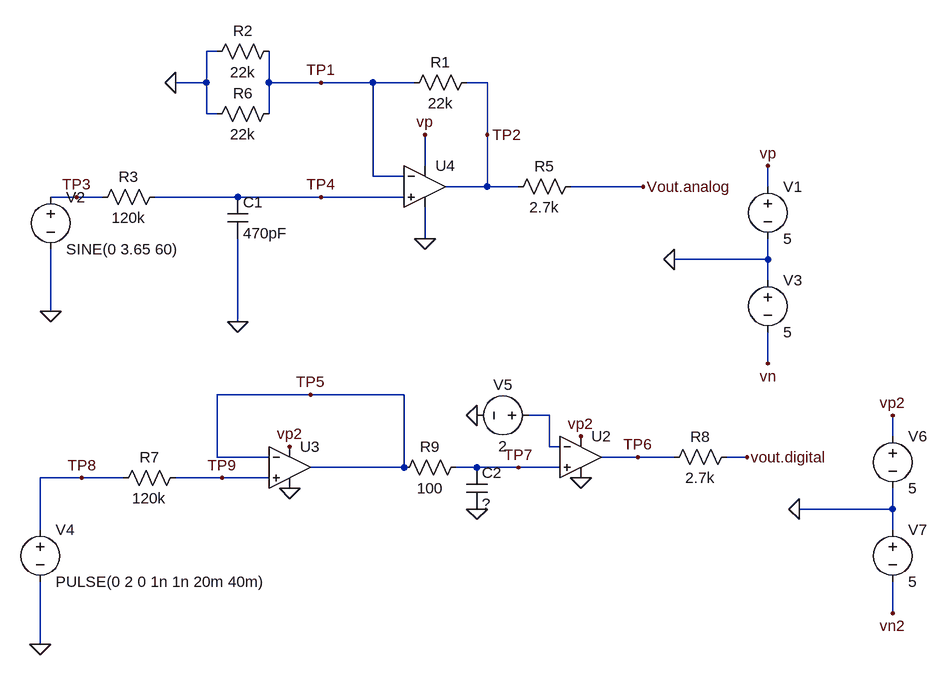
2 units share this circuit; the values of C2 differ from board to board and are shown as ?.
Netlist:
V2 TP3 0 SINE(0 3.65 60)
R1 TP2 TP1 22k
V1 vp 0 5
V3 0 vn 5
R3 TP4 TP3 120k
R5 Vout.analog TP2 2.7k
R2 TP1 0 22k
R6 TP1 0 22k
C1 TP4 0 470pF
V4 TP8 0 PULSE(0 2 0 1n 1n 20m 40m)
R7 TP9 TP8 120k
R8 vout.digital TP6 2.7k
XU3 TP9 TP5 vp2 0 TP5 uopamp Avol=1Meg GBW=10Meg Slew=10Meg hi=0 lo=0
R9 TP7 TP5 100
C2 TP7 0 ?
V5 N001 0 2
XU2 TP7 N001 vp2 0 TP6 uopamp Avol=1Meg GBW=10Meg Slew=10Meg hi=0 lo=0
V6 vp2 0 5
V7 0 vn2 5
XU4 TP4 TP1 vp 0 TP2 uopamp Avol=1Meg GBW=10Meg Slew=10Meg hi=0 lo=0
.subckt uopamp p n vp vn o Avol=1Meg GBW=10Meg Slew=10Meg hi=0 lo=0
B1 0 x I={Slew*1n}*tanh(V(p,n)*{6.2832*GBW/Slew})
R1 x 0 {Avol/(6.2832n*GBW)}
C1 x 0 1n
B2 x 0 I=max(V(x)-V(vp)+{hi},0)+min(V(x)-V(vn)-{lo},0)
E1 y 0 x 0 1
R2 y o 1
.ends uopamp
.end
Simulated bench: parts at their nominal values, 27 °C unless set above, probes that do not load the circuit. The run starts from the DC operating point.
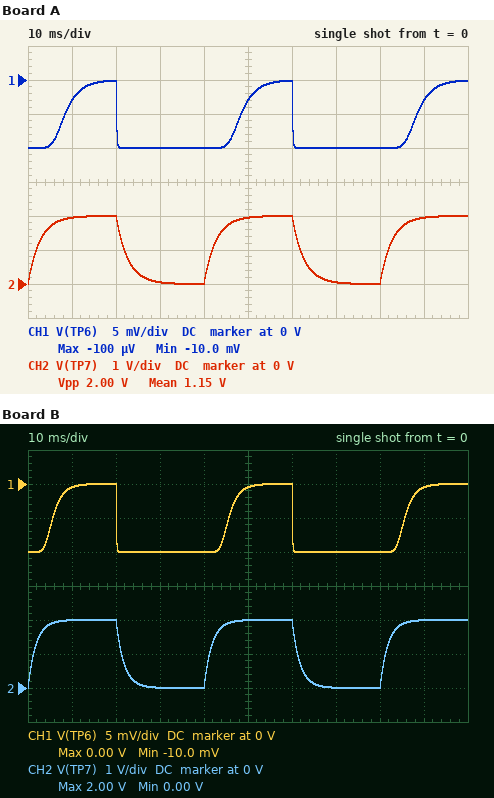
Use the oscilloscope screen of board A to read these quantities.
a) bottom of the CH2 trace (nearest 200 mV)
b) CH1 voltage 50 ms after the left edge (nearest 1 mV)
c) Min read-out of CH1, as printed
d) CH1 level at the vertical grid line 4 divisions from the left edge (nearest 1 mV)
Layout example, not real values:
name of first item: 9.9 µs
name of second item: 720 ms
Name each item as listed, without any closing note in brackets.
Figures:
bottom of the CH2 trace: 0 V
CH1 voltage 50 ms after the left edge: -3 mV
Min read-out of CH1, as printed: -10.0 mV
CH1 level at the vertical grid line 4 divisions from the left edge: -10 mV
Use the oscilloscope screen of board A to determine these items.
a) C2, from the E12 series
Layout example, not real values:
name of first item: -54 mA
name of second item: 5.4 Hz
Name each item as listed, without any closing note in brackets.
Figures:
C2, from the E12 series: 27 µF
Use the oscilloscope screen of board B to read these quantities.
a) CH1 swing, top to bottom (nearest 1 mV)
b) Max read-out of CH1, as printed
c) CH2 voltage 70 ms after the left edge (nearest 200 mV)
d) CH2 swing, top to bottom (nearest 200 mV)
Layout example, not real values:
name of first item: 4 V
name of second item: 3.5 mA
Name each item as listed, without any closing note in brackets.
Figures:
CH1 swing, top to bottom: 10 mV
Max read-out of CH1, as printed: 0.00 V
CH2 voltage 70 ms after the left edge: 0 V
CH2 swing, top to bottom: 2.0 V
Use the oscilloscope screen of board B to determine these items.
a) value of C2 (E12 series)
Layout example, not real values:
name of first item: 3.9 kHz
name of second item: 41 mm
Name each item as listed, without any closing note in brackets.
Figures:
value of C2: 18 µF
